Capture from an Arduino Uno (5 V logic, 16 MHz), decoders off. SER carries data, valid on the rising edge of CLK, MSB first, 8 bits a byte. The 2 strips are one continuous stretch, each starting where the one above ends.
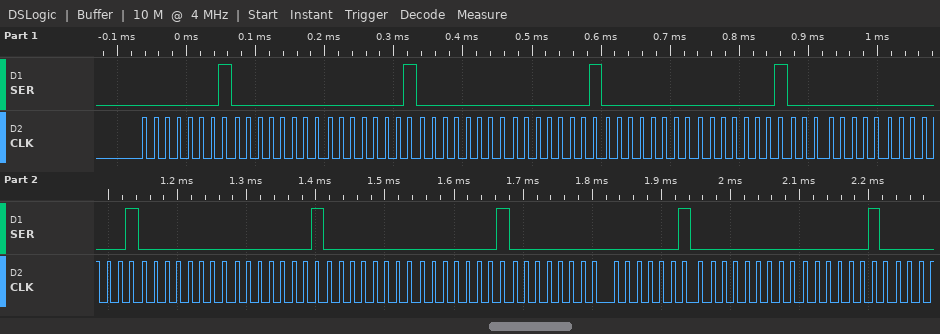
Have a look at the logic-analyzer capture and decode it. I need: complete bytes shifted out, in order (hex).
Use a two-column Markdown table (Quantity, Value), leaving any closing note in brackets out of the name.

| Quantity | Value |
|---|---|
| complete bytes shifted out, in order | 01 00 01 00 01 00 01 00 01 00 01 00 01 00 02 00 02 |
